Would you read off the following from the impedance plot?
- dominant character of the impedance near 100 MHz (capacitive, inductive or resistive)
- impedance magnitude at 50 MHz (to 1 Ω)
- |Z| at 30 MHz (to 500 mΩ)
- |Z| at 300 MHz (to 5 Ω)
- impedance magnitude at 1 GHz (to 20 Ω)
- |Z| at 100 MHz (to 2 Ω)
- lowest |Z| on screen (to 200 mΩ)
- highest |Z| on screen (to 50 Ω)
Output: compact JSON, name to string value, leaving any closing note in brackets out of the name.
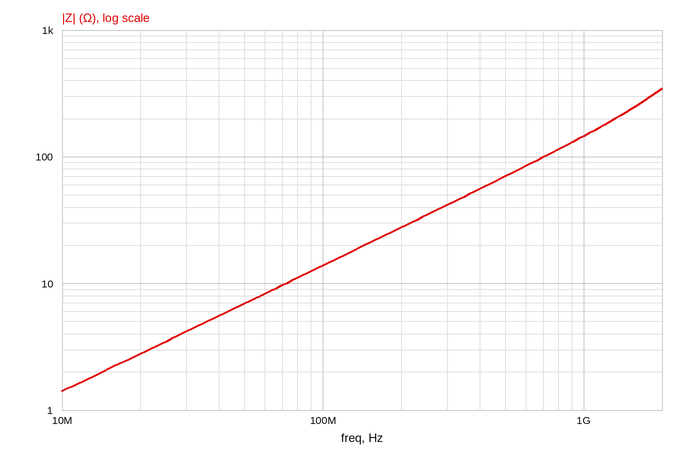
{"dominant character of the impedance near 100 MHz": "inductive", "impedance magnitude at 50 MHz": "7 Ω", "|Z| at 30 MHz": "4.0 Ω", "|Z| at 300 MHz": "40 Ω", "impedance magnitude at 1 GHz": "140 Ω", "|Z| at 100 MHz": "14 Ω", "lowest |Z| on screen": "1.4 Ω", "highest |Z| on screen": "350 Ω"}
